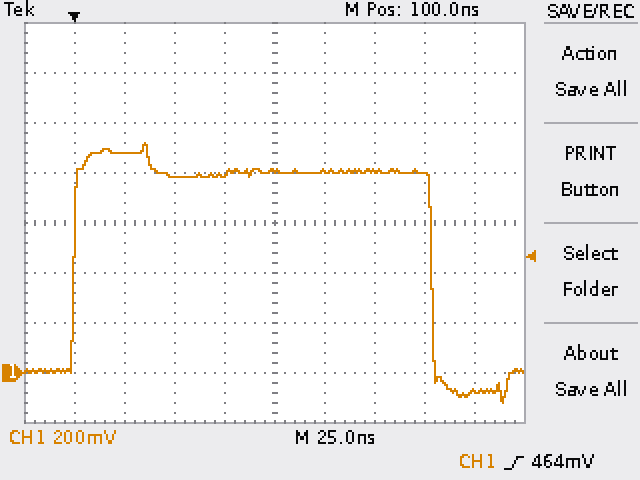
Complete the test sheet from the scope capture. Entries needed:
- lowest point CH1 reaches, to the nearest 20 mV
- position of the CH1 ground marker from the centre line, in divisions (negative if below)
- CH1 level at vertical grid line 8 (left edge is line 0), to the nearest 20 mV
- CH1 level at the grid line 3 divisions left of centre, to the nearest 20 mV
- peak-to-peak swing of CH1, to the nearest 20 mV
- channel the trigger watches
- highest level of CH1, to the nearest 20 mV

-120 mV
-3.0 div
800 mV
880 mV
1.04 V
CH1
920 mV
